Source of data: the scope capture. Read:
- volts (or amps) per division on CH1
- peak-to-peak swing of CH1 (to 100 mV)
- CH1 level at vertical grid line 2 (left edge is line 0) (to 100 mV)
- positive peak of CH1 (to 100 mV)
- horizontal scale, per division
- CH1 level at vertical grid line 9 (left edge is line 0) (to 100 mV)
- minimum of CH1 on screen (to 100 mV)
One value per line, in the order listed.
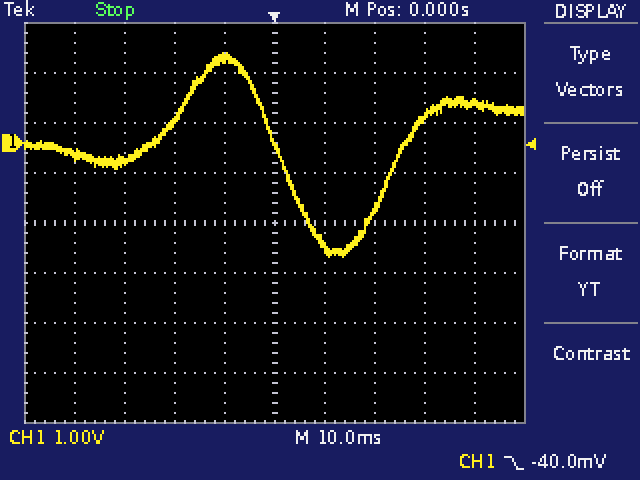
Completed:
1 V
4.1 V
-400 mV
1.8 V
10 ms
800 mV
-2.3 V
